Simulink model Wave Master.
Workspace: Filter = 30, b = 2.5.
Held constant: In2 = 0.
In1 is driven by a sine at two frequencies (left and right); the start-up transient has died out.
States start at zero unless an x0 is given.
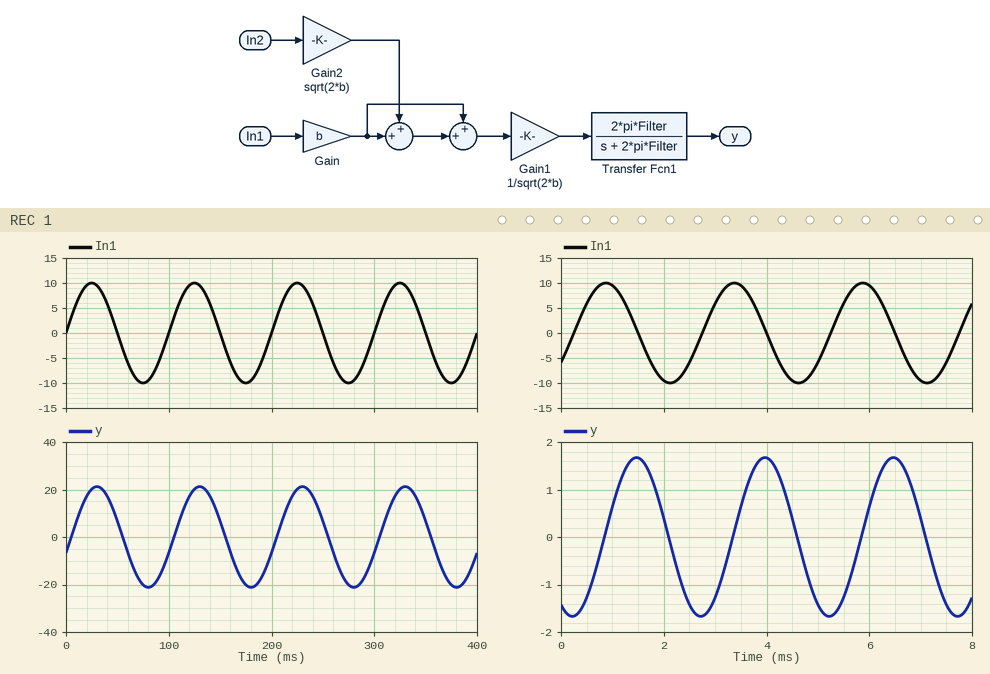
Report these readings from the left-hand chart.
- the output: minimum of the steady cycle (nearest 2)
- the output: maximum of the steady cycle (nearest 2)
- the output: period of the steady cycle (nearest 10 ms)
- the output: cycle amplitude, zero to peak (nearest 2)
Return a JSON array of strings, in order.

["-22", "22", "100 ms", "22"]
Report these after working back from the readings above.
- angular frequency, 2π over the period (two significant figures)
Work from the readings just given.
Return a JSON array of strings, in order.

["0.063 rad/ms"]
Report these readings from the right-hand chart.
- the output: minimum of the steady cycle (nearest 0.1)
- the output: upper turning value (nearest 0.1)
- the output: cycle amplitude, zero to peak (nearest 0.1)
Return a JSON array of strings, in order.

["-1.7", "1.7", "1.7"]
